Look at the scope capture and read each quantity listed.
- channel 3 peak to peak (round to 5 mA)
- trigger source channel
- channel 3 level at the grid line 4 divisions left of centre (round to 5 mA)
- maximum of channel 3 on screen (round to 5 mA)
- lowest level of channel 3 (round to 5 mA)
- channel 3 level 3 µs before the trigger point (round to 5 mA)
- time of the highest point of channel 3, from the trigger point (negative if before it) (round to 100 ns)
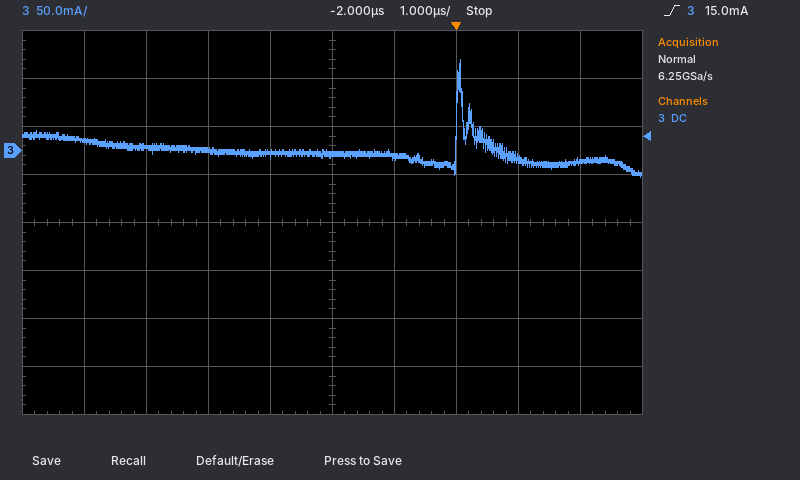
120 mA
channel 3
10 mA
95 mA
-25 mA
-5 mA
+100 ns
